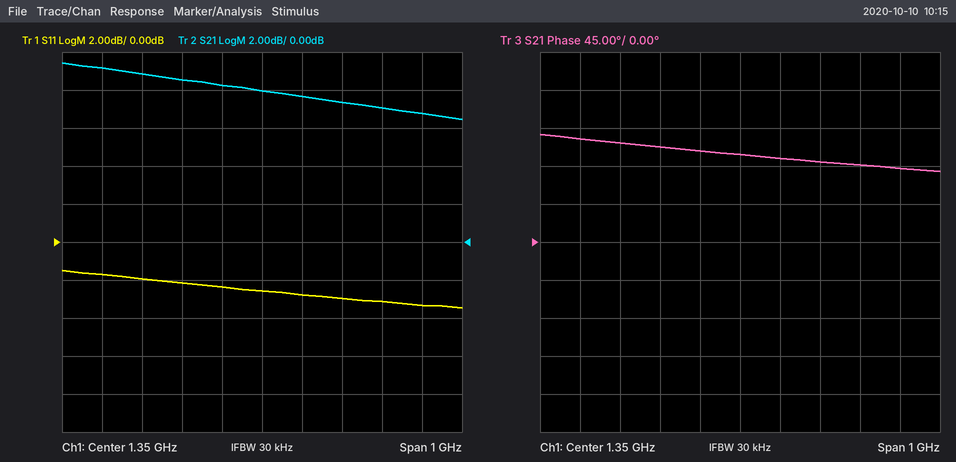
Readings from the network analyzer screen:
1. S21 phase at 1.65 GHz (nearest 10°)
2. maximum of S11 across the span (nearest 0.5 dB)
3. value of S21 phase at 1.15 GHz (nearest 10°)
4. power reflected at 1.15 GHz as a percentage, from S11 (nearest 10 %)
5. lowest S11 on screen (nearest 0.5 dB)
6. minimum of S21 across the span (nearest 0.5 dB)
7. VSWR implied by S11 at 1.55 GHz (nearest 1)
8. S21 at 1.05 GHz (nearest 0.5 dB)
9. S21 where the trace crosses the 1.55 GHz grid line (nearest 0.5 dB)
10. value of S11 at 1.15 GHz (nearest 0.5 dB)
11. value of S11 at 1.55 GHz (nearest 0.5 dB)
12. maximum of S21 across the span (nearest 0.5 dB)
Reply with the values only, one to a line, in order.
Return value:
90°
-1.5 dB
110°
60 %
-3.5 dB
6.5 dB
6
9.0 dB
7.5 dB
-2.0 dB
-3.0 dB
9.5 dB
